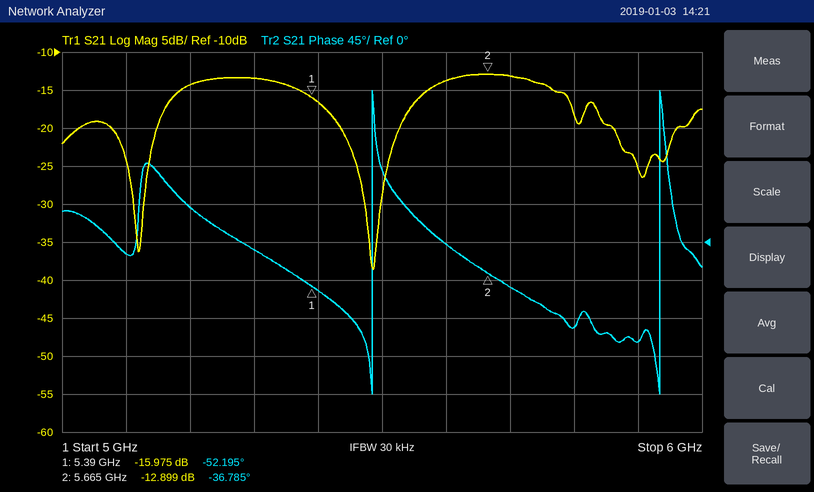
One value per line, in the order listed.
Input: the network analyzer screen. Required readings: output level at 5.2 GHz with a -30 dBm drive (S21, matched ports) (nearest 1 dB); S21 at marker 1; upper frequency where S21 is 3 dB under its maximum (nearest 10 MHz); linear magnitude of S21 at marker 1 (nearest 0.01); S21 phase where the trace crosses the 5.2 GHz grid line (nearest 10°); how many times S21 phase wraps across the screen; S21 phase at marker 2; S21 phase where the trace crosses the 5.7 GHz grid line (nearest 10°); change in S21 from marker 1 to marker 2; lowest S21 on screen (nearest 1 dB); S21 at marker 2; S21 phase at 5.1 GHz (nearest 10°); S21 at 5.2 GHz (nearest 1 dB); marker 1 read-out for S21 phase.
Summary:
-44 dBm
-15.975 dB
5.79 GHz
0.16
40°
2
-36.785°
-50°
3.076 dB
-39 dB
-12.899 dB
-10°
-14 dB
-52.195°
